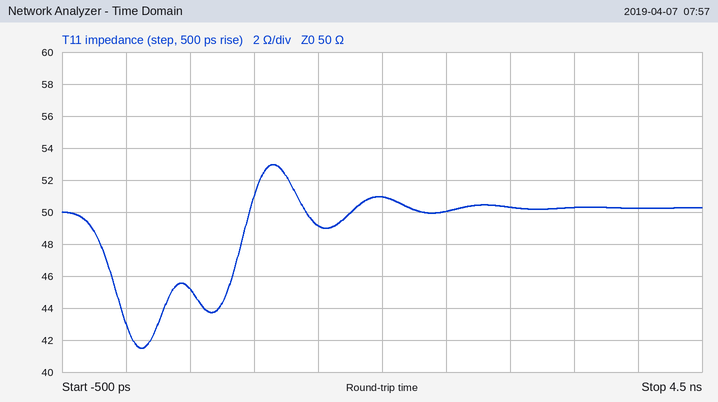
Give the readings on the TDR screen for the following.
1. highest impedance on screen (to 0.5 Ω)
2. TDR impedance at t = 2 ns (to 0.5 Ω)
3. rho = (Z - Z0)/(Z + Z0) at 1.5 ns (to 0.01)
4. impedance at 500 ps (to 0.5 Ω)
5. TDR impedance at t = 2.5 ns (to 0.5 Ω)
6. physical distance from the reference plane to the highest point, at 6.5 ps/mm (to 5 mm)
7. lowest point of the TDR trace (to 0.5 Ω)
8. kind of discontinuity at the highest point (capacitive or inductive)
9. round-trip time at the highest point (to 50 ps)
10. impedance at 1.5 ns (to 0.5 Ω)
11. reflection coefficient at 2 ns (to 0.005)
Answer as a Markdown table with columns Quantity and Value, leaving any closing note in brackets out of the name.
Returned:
| Quantity | Value |
|---|---|
| highest impedance on screen | 53.0 Ω |
| TDR impedance at t = 2 ns | 51.0 Ω |
| rho = (Z - Z0)/(Z + Z0) at 1.5 ns | -0.01 |
| impedance at 500 ps | 45.0 Ω |
| TDR impedance at t = 2.5 ns | 50.0 Ω |
| physical distance from the reference plane to the highest point, at 6.5 ps/mm | 90 mm |
| lowest point of the TDR trace | 41.5 Ω |
| kind of discontinuity at the highest point | inductive |
| round-trip time at the highest point | 1.15 ns |
| impedance at 1.5 ns | 49.0 Ω |
| reflection coefficient at 2 ns | +0.010 |
